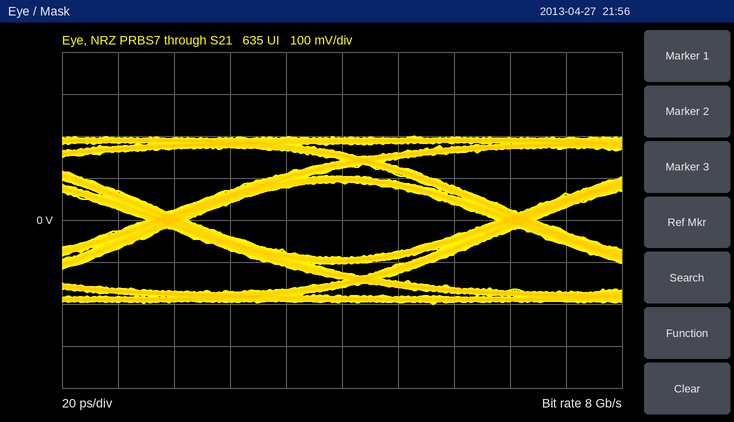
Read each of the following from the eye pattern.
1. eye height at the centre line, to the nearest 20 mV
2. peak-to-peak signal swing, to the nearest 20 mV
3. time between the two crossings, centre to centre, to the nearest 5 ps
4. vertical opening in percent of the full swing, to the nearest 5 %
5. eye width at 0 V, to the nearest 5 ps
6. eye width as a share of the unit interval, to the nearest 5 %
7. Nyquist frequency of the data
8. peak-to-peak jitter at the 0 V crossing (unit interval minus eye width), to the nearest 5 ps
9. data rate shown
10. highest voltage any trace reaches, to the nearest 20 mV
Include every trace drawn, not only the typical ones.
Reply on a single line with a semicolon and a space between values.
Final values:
180 mV; 400 mV; 125 ps; 45 %; 110 ps; 90 %; 4 GHz; 15 ps; 8 Gb/s; 200 mV
